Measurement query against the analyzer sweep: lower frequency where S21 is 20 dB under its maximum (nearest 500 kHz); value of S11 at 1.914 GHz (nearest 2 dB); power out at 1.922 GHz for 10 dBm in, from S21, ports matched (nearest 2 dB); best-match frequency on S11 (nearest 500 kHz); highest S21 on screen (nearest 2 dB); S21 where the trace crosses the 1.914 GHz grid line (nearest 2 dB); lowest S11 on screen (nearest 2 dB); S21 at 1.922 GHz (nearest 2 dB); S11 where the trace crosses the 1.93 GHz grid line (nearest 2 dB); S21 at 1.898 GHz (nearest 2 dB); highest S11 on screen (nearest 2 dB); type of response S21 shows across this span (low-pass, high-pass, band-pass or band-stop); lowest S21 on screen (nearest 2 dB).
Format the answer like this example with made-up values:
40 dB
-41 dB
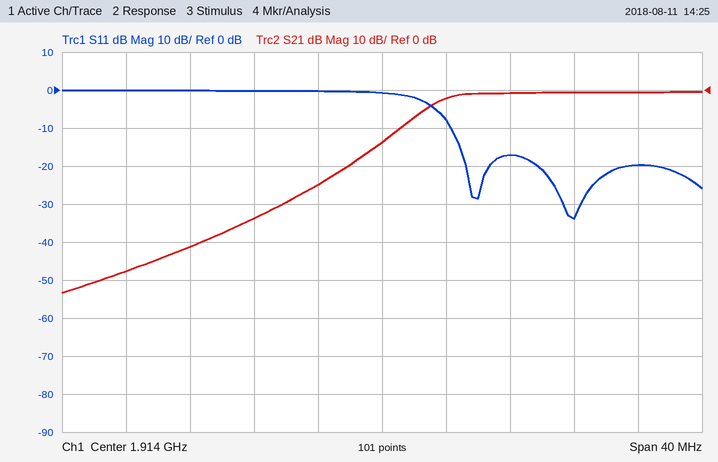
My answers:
1.9115 GHz
0 dB
10 dBm
1.9260 GHz
0 dB
-14 dB
-34 dB
0 dB
-20 dB
-48 dB
0 dB
high-pass
-54 dB
